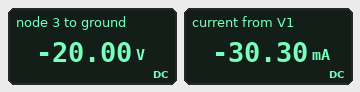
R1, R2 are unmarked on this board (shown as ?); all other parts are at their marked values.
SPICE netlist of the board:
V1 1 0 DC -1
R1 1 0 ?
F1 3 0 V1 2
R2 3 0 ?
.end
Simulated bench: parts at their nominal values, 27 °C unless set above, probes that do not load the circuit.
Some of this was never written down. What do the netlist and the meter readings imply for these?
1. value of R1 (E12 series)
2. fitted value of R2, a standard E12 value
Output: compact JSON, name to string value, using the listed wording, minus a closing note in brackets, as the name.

{"value of R1": "33 Ω", "fitted value of R2, a standard E12 value": "330 Ω"}
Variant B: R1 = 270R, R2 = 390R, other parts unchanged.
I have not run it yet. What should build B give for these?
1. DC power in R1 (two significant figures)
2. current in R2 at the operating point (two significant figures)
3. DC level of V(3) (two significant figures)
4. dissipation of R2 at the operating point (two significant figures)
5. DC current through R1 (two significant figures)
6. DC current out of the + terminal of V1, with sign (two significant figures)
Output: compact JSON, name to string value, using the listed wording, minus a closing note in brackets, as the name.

{"DC power in R1": "3.7 mW", "current in R2 at the operating point": "7.4 mA", "DC level of V(3)": "-2.9 V", "dissipation of R2 at the operating point": "21 mW", "DC current through R1": "3.7 mA", "DC current out of the + terminal of V1, with sign": "-3.7 mA"}
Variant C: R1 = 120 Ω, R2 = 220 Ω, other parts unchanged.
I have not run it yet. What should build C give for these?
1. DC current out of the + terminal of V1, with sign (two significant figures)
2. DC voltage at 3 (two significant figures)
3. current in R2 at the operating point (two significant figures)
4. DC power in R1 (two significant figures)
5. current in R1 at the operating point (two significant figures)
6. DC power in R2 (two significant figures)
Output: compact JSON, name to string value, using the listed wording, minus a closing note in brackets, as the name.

{"DC current out of the + terminal of V1, with sign": "-8.3 mA", "DC voltage at 3": "-3.7 V", "current in R2 at the operating point": "17 mA", "DC power in R1": "8.3 mW", "current in R1 at the operating point": "8.3 mA", "DC power in R2": "61 mW"}
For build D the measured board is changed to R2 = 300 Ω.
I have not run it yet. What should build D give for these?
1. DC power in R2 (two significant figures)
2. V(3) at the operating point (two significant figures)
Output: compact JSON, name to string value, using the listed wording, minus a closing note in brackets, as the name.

{"DC power in R2": "1.1 W", "V(3) at the operating point": "-18 V"}
